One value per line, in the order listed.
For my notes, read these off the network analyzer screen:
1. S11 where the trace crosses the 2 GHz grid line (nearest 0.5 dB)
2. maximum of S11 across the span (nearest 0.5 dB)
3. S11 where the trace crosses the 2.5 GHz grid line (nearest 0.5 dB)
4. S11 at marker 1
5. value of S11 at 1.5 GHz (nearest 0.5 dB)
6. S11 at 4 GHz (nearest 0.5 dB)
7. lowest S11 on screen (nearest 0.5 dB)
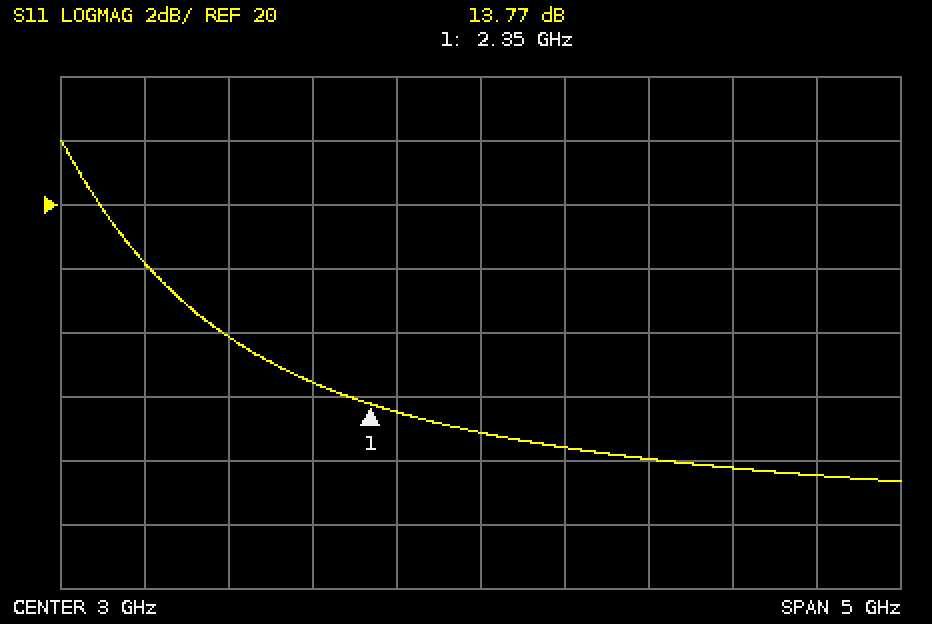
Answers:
14.5 dB
22.0 dB
13.5 dB
13.77 dB
16.0 dB
12.0 dB
11.5 dB
